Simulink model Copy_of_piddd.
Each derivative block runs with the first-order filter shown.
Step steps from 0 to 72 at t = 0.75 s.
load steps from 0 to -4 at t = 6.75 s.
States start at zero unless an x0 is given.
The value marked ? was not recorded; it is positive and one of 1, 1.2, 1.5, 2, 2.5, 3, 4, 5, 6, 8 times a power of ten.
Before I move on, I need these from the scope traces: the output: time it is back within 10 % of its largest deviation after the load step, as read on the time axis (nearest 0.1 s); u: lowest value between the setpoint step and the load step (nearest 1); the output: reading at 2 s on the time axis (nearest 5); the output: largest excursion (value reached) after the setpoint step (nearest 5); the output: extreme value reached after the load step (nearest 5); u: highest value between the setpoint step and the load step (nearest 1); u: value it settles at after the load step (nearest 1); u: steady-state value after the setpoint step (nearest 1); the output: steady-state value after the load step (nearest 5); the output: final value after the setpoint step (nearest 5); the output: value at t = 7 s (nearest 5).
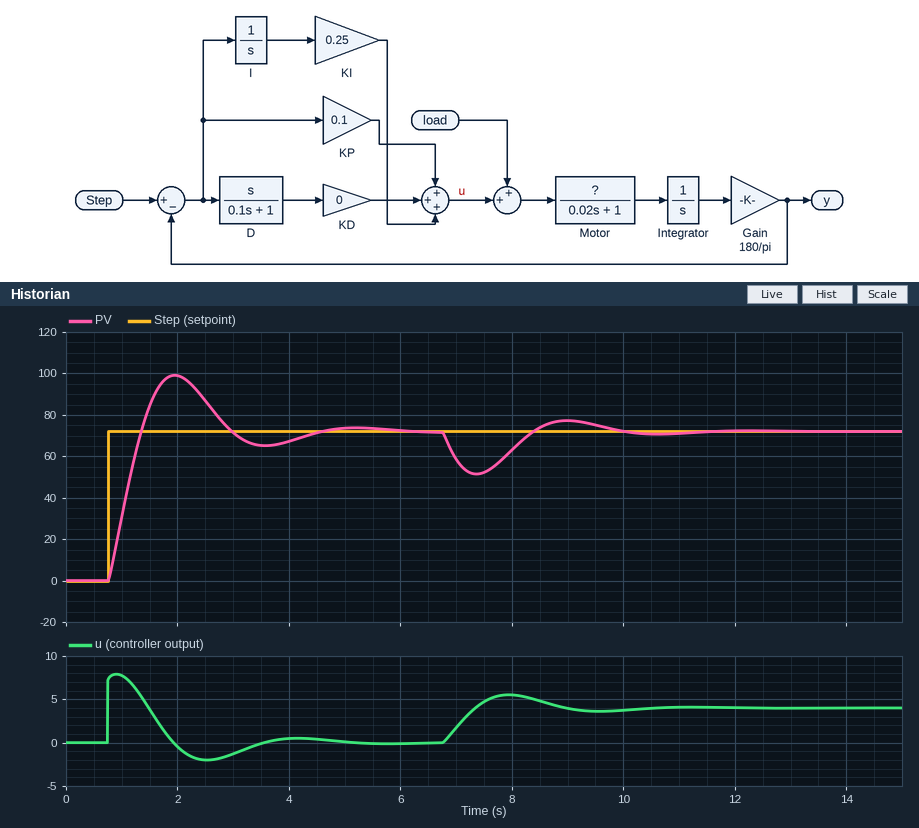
9.7 s
-2
100
100
50
8
4
0
70
70
60
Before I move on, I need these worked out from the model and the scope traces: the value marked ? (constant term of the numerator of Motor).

0.3
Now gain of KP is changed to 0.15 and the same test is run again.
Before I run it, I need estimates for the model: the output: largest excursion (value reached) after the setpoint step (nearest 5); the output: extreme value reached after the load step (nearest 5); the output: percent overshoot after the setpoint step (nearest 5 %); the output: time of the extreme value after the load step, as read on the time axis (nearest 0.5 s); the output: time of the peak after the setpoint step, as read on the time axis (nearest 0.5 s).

90
55
25 %
7.5 s
2.0 s
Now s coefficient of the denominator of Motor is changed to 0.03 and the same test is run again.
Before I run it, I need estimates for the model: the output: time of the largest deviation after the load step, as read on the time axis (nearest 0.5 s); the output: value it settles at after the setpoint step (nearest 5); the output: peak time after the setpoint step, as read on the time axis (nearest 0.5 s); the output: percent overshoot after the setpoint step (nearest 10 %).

7.5 s
70
2.0 s
40 %
